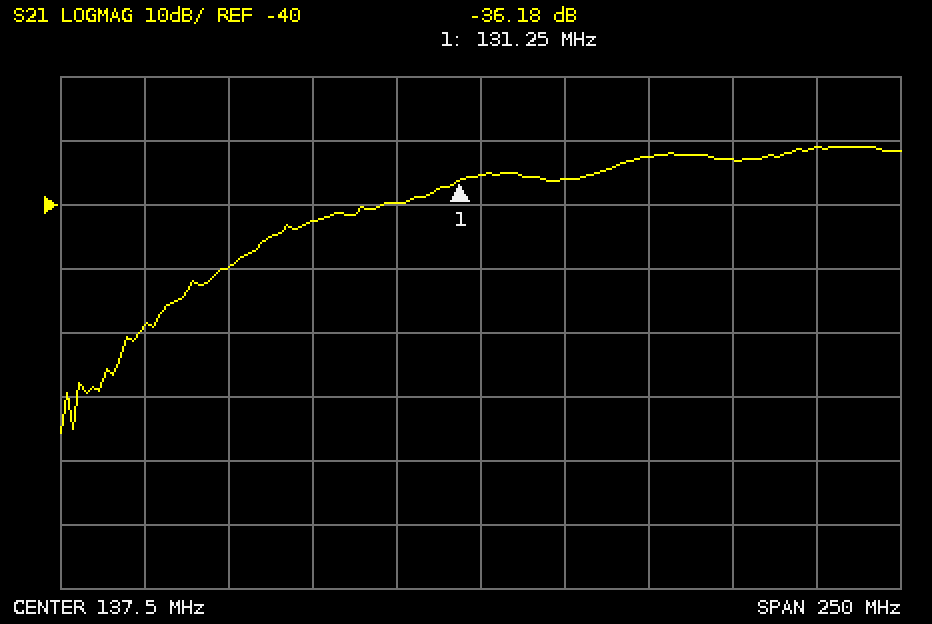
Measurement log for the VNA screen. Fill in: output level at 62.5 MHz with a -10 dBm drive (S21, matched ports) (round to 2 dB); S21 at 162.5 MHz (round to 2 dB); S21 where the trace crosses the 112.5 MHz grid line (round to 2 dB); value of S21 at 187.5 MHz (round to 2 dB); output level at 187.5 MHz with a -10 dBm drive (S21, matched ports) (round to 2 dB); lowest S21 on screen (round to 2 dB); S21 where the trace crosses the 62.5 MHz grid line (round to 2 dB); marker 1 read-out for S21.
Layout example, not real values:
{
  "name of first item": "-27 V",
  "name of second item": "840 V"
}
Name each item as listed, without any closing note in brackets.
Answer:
{
  "output level at 62.5 MHz with a -10 dBm drive (S21, matched ports)": "-60 dBm",
  "S21 at 162.5 MHz": "-36 dB",
  "S21 where the trace crosses the 112.5 MHz grid line": "-40 dB",
  "value of S21 at 187.5 MHz": "-32 dB",
  "output level at 187.5 MHz with a -10 dBm drive (S21, matched ports)": "-42 dBm",
  "lowest S21 on screen": "-76 dB",
  "S21 where the trace crosses the 62.5 MHz grid line": "-50 dB",
  "marker 1 read-out for S21": "-36.18 dB"
}
